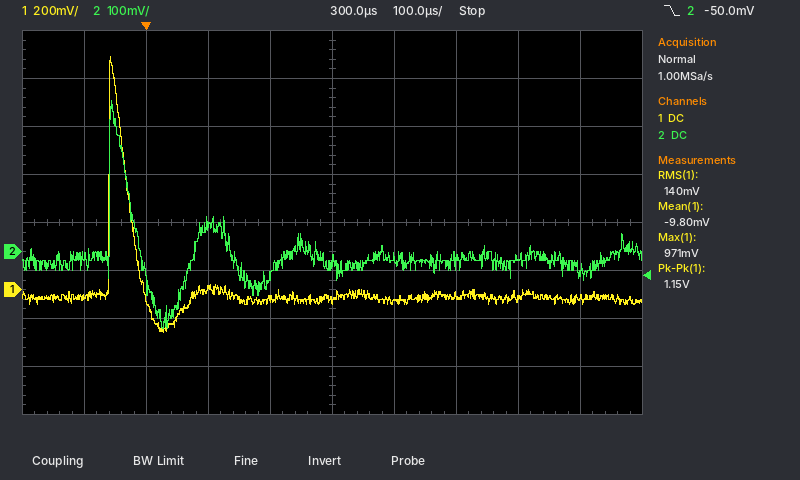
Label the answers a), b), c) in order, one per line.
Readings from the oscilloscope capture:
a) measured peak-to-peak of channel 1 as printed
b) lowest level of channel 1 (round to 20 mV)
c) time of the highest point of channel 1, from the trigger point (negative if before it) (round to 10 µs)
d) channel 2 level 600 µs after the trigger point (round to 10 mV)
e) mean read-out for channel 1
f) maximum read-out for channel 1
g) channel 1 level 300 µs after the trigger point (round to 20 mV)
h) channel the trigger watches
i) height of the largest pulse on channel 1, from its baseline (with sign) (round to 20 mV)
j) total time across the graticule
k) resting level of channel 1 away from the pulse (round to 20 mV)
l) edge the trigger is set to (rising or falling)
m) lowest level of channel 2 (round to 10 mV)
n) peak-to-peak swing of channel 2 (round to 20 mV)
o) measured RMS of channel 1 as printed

a) 1.15 V
b) -180 mV
c) -60 µs
d) -10 mV
e) -9.80 mV
f) 971 mV
g) -40 mV
h) channel 2
i) +1.00 V
j) 1 ms
k) -40 mV
l) falling
m) -160 mV
n) 480 mV
o) 140 mV
